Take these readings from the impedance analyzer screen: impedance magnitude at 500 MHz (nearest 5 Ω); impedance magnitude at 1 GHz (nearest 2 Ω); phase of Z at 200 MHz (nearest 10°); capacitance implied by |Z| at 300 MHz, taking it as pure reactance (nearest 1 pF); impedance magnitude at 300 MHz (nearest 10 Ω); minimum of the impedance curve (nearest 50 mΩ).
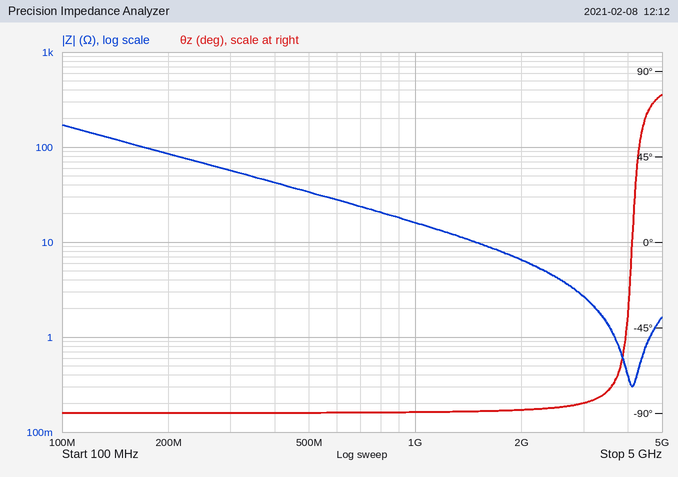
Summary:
35 Ω
16 Ω
-90°
9 pF
60 Ω
300 mΩ
